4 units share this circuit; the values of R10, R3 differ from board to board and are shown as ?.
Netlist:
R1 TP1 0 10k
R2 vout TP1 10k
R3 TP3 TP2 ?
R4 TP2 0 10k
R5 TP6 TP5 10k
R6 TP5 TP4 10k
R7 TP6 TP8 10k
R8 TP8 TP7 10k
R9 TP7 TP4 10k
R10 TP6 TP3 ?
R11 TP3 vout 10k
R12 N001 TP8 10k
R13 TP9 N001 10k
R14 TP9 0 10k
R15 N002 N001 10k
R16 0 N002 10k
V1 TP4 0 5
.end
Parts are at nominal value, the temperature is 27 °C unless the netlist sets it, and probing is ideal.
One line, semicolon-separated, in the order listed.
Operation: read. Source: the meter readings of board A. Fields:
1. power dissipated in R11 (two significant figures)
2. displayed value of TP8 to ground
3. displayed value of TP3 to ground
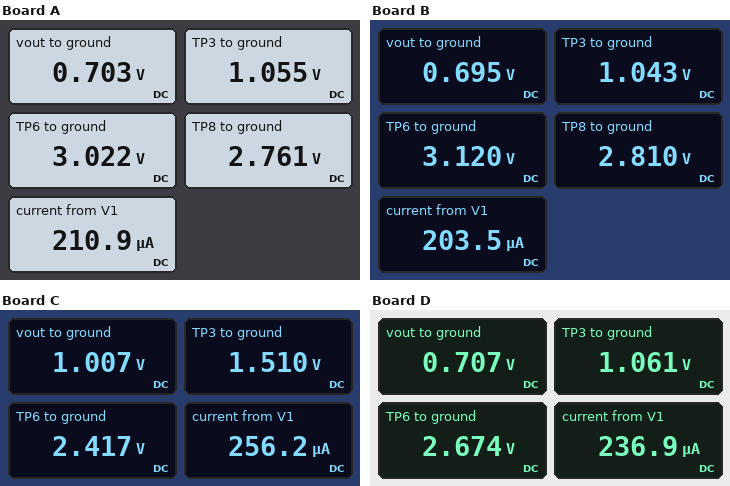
12 µW; 2.761 V; 1.055 V
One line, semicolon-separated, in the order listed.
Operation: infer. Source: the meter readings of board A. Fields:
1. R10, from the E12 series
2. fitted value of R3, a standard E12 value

27 kΩ; 18 kΩ
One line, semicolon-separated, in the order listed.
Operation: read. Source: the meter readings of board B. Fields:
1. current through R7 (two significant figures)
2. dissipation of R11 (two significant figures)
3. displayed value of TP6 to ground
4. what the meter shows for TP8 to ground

31 µA; 12 µW; 3.120 V; 2.810 V
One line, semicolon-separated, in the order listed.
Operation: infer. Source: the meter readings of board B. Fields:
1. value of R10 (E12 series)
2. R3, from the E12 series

33 kΩ; 27 kΩ
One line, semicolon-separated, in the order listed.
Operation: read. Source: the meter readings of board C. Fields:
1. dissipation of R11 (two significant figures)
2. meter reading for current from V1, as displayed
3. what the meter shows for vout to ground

25 µW; 256.2 µA; 1.007 V
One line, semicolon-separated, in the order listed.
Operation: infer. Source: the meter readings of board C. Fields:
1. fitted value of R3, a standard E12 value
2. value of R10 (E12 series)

8.2 kΩ; 6.8 kΩ
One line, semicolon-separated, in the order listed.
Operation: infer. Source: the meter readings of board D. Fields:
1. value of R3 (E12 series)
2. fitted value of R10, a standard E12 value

4.7 kΩ; 15 kΩ
